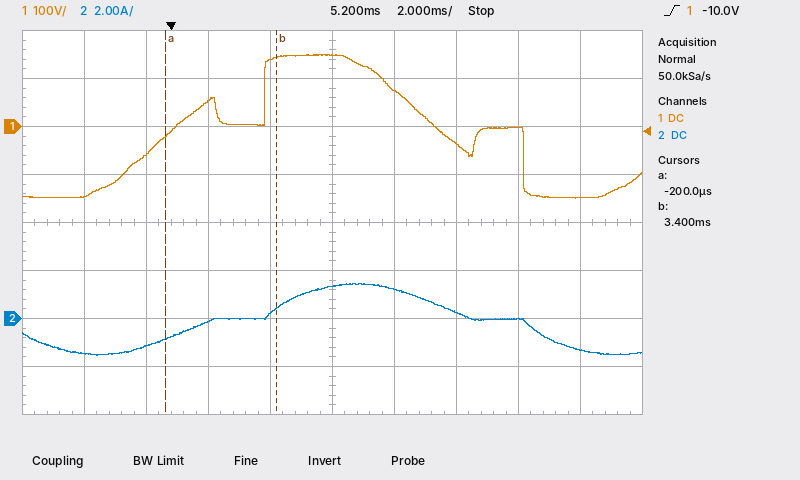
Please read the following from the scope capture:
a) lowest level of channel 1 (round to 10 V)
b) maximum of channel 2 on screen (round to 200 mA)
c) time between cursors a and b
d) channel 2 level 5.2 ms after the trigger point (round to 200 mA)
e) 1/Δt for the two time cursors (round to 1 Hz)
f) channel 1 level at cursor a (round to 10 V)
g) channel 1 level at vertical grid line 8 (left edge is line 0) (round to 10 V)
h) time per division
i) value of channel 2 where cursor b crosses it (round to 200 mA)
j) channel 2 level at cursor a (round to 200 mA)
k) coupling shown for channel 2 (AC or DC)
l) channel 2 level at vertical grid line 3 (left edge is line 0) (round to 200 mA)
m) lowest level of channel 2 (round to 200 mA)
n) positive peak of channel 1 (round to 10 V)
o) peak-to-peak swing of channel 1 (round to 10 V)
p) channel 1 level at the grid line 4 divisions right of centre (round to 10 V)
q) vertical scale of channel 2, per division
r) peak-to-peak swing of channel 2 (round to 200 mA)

-150 V
1.4 A
3.6 ms
1.4 A
278 Hz
-20 V
0 V
2 ms
400 mA
-800 mA
DC
-200 mA
-1.6 A
150 V
300 V
-150 V
2 A
3.0 A
